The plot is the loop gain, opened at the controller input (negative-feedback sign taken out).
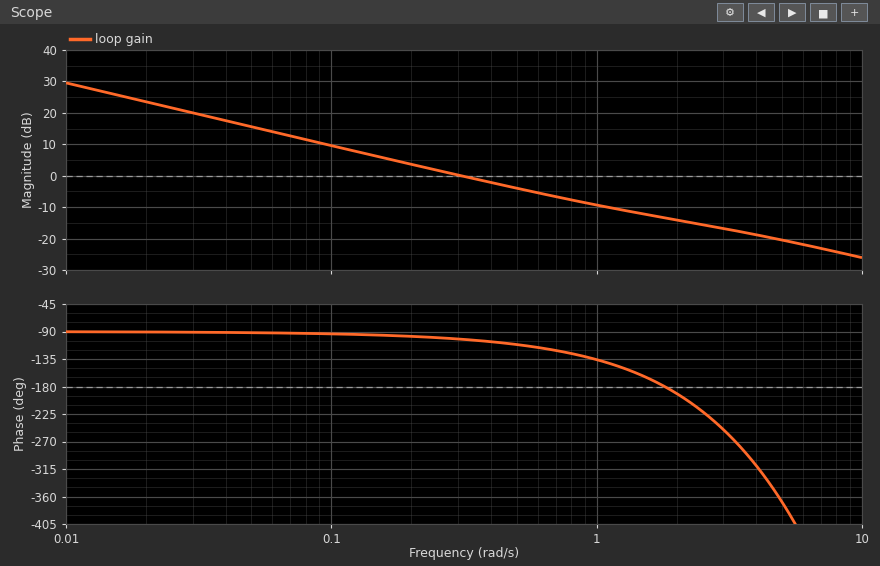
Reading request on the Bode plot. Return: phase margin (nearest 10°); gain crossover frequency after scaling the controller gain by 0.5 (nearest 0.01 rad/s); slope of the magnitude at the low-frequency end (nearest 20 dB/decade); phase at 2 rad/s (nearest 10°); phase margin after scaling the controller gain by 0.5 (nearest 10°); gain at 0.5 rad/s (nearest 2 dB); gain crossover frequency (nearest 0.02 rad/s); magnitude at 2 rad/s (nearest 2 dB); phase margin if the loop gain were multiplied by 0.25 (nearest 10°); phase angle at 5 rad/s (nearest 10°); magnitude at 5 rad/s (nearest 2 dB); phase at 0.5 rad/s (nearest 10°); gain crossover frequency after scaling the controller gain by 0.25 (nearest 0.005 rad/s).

80°
0.15 rad/s
-20 dB/decade
-190°
80°
-4 dB
0.30 rad/s
-14 dB
90°
-370°
-20 dB
-110°
0.075 rad/s
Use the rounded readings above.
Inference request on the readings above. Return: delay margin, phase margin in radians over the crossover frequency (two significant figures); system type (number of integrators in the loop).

4.7 s
1
